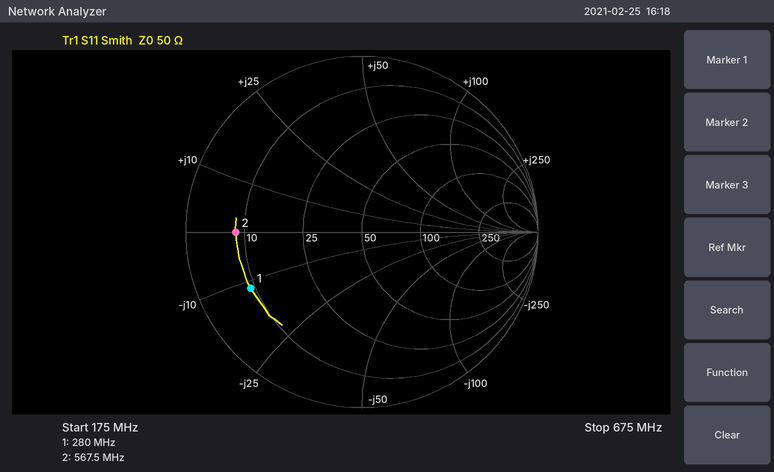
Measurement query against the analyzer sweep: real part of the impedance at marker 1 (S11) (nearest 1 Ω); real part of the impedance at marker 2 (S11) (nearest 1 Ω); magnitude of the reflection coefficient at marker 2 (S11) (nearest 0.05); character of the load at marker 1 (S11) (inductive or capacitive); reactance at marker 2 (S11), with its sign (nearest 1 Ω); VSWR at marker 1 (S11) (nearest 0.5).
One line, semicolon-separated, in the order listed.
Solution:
9 Ω; 8 Ω; 0.70; capacitive; 0 Ω; 6.0
